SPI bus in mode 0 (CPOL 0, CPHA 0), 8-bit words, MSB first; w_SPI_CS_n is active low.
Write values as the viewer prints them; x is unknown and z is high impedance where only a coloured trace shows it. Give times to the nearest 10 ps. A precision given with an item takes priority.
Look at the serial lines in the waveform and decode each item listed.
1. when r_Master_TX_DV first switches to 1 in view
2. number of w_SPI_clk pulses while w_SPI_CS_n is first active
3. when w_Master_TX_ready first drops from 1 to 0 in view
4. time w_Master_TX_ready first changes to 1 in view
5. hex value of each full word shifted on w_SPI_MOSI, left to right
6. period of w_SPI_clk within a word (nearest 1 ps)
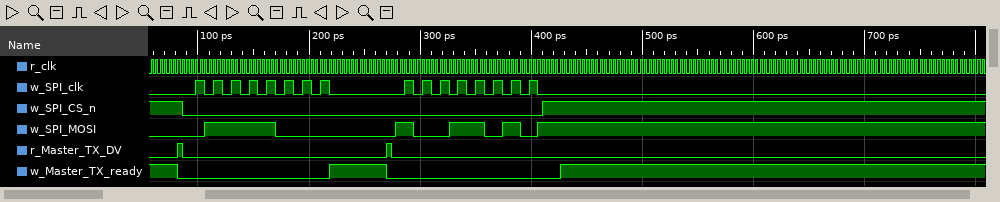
80 ps
16
80 ps
220 ps
78, 9A
16 ps
